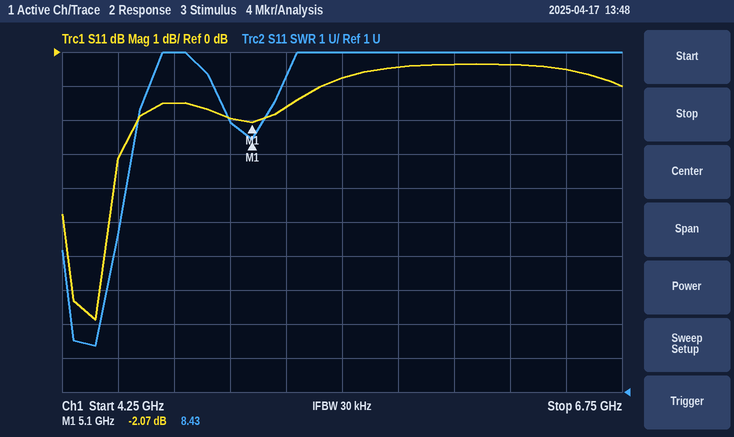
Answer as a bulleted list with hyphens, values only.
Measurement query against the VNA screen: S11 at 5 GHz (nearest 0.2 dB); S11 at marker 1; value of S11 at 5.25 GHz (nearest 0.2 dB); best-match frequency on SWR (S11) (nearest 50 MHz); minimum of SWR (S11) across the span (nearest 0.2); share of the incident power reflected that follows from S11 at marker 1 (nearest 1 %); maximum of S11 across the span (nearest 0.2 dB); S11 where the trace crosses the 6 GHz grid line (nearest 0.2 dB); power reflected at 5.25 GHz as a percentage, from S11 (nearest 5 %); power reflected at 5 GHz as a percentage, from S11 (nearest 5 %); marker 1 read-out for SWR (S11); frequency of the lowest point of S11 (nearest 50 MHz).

- -2.0 dB
- -2.07 dB
- -1.6 dB
- 4.40 GHz
- 2.4
- 62 %
- -0.4 dB
- -0.4 dB
- 70 %
- 65 %
- 8.43
- 4.40 GHz
